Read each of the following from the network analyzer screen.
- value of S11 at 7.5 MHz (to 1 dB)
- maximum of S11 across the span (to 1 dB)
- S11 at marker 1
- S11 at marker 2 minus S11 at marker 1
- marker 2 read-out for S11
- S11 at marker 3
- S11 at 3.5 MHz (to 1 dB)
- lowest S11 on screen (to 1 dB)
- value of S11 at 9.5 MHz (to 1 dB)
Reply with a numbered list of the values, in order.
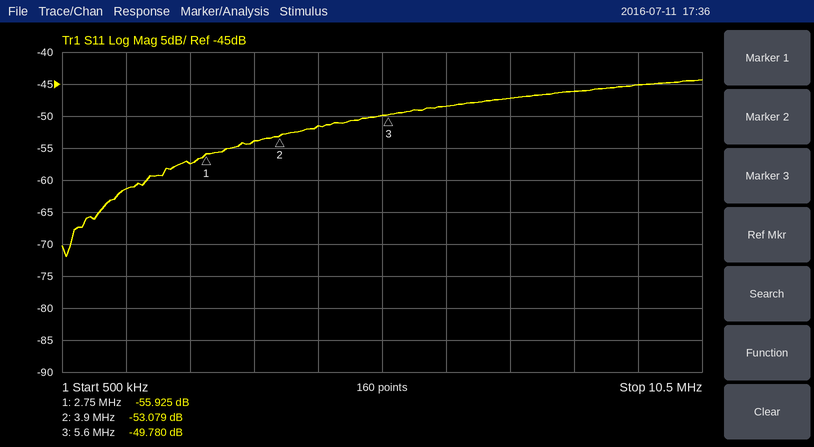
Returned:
1. -47 dB
2. -44 dB
3. -55.925 dB
4. 2.846 dB
5. -53.079 dB
6. -49.780 dB
7. -54 dB
8. -72 dB
9. -45 dB
